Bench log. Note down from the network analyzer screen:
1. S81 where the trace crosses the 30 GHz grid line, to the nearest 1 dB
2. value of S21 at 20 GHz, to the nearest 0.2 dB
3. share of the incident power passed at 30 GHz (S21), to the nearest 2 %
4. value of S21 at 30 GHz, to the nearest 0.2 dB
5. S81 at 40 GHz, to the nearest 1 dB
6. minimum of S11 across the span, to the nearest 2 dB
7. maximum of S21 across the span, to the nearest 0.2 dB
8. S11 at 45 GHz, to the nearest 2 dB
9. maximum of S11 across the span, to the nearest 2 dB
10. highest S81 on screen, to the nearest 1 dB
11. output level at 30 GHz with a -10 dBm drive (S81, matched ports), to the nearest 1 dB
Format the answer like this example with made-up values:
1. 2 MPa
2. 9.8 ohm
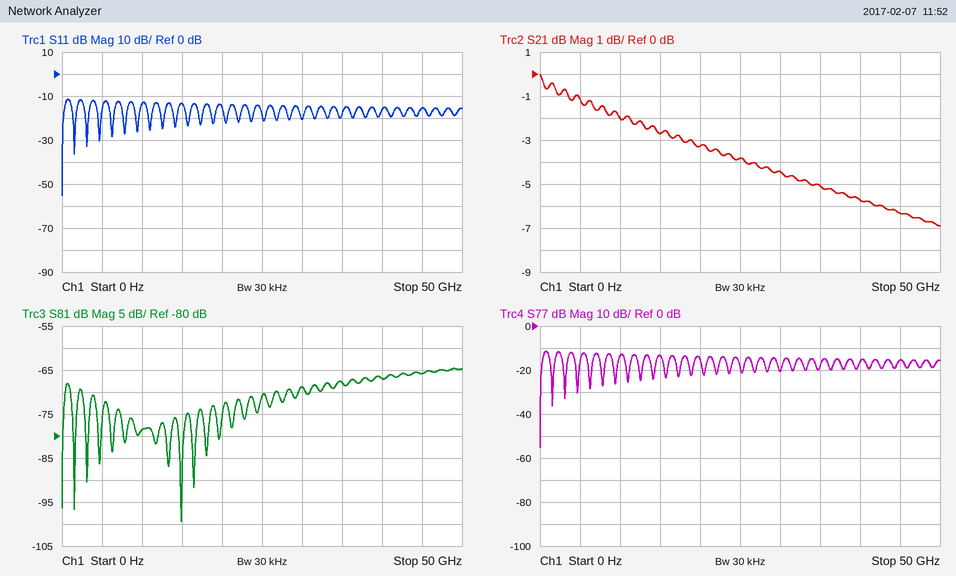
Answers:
1. -69 dB
2. -3.2 dB
3. 36 %
4. -4.4 dB
5. -67 dB
6. -56 dB
7. 0.0 dB
8. -16 dB
9. -12 dB
10. -65 dB
11. -79 dBm
